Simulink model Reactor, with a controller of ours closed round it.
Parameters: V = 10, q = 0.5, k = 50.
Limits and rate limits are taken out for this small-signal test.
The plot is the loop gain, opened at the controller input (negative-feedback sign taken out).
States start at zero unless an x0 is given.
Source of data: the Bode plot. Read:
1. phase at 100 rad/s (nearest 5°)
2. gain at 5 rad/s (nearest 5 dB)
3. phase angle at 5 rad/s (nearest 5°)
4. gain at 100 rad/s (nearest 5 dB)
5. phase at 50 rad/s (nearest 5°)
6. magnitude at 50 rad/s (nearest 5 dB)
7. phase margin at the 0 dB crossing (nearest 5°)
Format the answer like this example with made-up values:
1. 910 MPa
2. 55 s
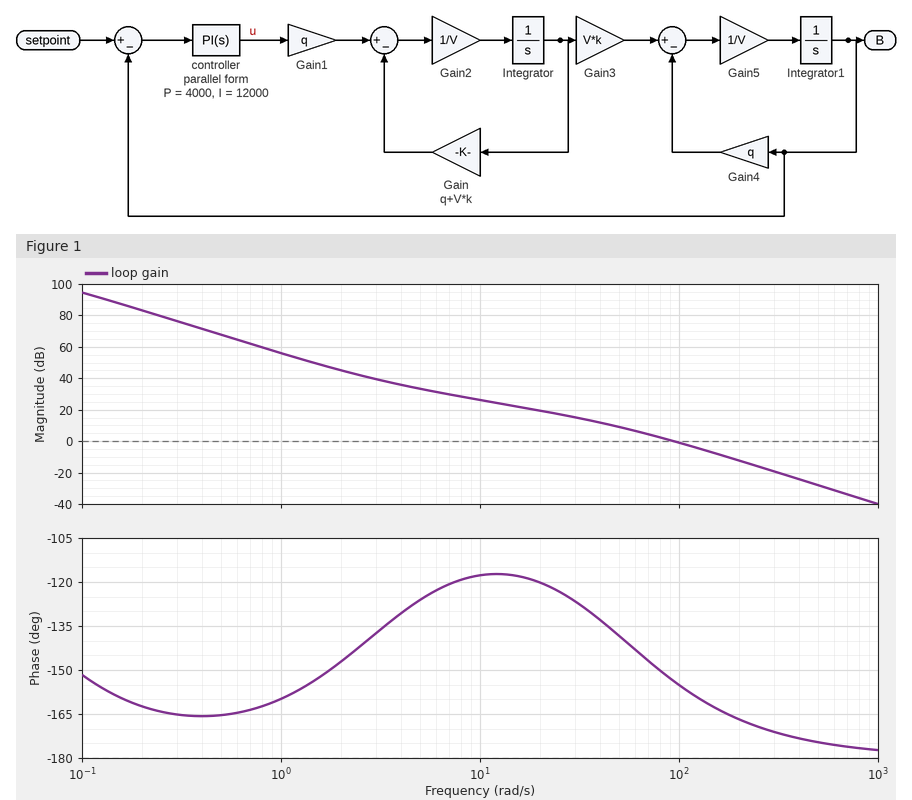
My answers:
1. -155°
2. 35 dB
3. -125°
4. 0 dB
5. -140°
6. 10 dB
7. 25°
